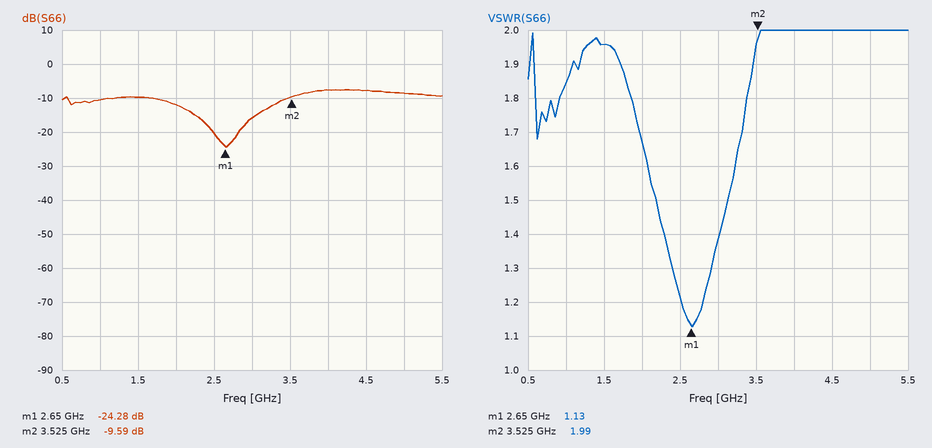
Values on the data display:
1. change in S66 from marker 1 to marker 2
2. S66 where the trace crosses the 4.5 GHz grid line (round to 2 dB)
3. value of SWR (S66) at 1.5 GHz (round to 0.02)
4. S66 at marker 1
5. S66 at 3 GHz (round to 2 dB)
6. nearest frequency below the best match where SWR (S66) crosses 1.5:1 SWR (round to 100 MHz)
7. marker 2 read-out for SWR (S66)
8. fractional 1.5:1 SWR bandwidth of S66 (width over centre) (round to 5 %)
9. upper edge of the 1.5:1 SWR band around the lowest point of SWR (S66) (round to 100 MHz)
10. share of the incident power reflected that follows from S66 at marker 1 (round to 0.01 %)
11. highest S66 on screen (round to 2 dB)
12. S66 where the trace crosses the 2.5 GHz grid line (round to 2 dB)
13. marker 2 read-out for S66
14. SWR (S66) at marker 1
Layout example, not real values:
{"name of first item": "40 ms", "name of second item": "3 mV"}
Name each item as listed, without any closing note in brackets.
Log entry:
{"change in S66 from marker 1 to marker 2": "14.69 dB", "S66 where the trace crosses the 4.5 GHz grid line": "-8 dB", "value of SWR (S66) at 1.5 GHz": "1.96", "S66 at marker 1": "-24.28 dB", "S66 at 3 GHz": "-16 dB", "nearest frequency below the best match where SWR (S66) crosses 1.5:1 SWR": "2.2 GHz", "marker 2 read-out for SWR": "1.99", "fractional 1.5:1 SWR bandwidth of S66 (width over centre)": "35 %", "upper edge of the 1.5:1 SWR band around the lowest point of SWR (S66)": "3.1 GHz", "share of the incident power reflected that follows from S66 at marker 1": "0.37 %", "highest S66 on screen": "-8 dB", "S66 where the trace crosses the 2.5 GHz grid line": "-20 dB", "marker 2 read-out for S66": "-9.59 dB", "SWR (S66) at marker 1": "1.13"}
